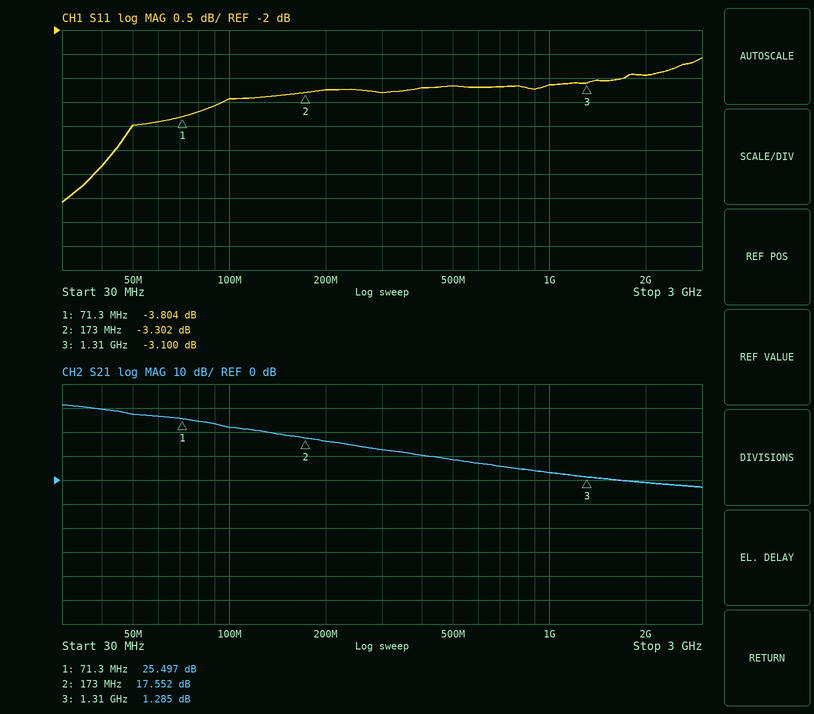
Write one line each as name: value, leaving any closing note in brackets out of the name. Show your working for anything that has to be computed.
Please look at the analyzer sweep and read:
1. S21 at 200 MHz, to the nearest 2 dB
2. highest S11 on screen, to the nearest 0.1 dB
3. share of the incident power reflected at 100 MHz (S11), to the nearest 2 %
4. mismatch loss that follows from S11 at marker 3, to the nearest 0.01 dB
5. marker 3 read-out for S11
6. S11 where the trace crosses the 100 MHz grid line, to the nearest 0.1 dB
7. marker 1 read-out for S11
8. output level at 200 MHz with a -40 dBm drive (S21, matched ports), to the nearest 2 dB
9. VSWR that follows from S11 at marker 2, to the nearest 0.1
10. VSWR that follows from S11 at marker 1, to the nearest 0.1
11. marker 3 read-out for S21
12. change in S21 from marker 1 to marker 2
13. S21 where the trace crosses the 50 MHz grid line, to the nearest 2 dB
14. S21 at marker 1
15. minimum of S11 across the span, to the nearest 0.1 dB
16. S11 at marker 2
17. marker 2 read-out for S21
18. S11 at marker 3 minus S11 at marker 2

S21 at 200 MHz, to the nearest 2 dB: 16 dB
highest S11 on screen, to the nearest 0.1 dB: -2.6 dB
share of the incident power reflected at 100 MHz (S11), to the nearest 2 %: 10^(-3.4/10) ≈ 46 %
mismatch loss that follows from S11 at marker 3, to the nearest 0.01 dB: −10 log10(1 − 10^(-3.1/10)) ≈ 2.92 dB
marker 3 read-out for S11: -3.100 dB
S11 where the trace crosses the 100 MHz grid line, to the nearest 0.1 dB: -3.4 dB
marker 1 read-out for S11: -3.804 dB
output level at 200 MHz with a -40 dBm drive (S21, matched ports), to the nearest 2 dB: -40 dBm + (16 dB) = -24 dBm
VSWR that follows from S11 at marker 2, to the nearest 0.1: (1 + 0.6838)/(1 − 0.6838) ≈ 5.3
VSWR that follows from S11 at marker 1, to the nearest 0.1: (1 + 0.6454)/(1 − 0.6454) ≈ 4.6
marker 3 read-out for S21: 1.285 dB
change in S21 from marker 1 to marker 2: 17.552 − (25.497) = -7.945 dB
S21 where the trace crosses the 50 MHz grid line, to the nearest 2 dB: 28 dB
S21 at marker 1: 25.497 dB
minimum of S11 across the span, to the nearest 0.1 dB: -5.6 dB
S11 at marker 2: -3.302 dB
marker 2 read-out for S21: 17.552 dB
S11 at marker 3 minus S11 at marker 2: -3.1 − (-3.302) = 0.202 dB
